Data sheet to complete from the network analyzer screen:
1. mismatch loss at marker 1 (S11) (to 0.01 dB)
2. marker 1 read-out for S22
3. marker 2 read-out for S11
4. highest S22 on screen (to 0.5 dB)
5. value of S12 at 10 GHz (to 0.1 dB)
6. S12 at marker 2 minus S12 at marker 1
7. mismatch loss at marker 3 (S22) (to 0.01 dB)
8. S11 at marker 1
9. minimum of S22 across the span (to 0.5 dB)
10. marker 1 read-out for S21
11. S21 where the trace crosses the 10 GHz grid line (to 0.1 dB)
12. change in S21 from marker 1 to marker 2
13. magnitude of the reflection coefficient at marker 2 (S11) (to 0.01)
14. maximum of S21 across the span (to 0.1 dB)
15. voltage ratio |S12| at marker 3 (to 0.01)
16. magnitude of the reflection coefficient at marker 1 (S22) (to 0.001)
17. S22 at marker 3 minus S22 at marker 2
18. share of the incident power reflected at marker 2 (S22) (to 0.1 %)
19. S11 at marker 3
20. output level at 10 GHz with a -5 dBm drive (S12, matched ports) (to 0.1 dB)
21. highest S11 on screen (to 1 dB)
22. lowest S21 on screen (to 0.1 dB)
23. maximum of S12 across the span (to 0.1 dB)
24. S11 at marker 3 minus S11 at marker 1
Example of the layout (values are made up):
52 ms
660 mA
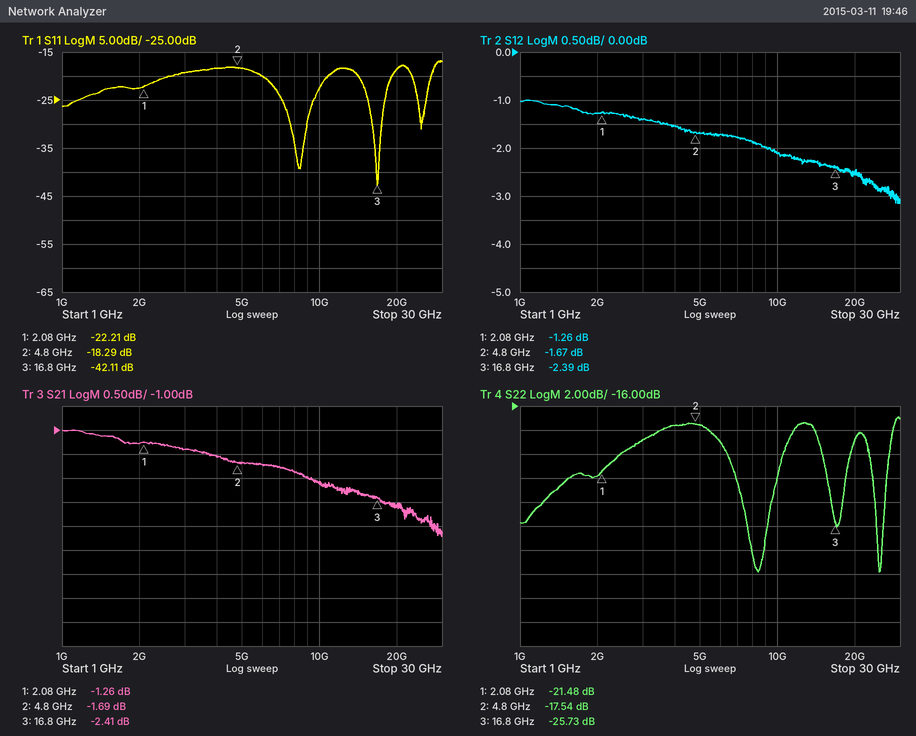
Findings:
0.03 dB
-21.48 dB
-18.29 dB
-17.0 dB
-2.1 dB
-0.41 dB
0.01 dB
-22.21 dB
-30.0 dB
-1.26 dB
-2.1 dB
-0.43 dB
0.12
-1.0 dB
0.76
0.084
-8.19 dB
1.8 %
-42.11 dB
-7.1 dBm
-17 dB
-3.2 dB
-1.0 dB
-19.90 dB
